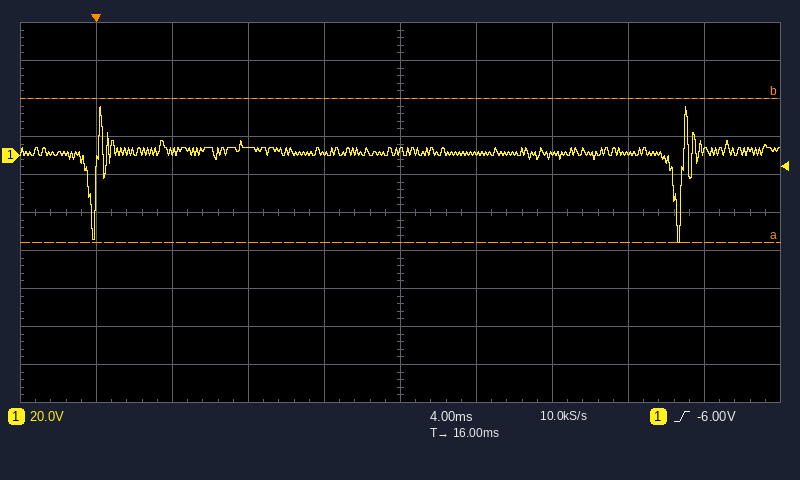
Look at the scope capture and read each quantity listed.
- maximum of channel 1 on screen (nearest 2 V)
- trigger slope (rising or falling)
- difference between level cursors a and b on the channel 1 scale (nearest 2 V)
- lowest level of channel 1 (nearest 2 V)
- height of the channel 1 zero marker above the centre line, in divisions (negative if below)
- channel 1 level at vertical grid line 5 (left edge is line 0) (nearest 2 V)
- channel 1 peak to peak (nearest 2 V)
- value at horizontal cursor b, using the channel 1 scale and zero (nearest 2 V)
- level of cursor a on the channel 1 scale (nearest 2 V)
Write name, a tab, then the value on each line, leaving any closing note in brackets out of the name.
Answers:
maximum of channel 1 on screen	26 V
trigger slope	rising
difference between level cursors a and b on the channel 1 scale	76 V
lowest level of channel 1	-46 V
height of the channel 1 zero marker above the centre line, in divisions	+1.5 div
channel 1 level at vertical grid line 5 (left edge is line 0)	2 V
channel 1 peak to peak	72 V
value at horizontal cursor b, using the channel 1 scale and zero	30 V
level of cursor a on the channel 1 scale	-46 V
